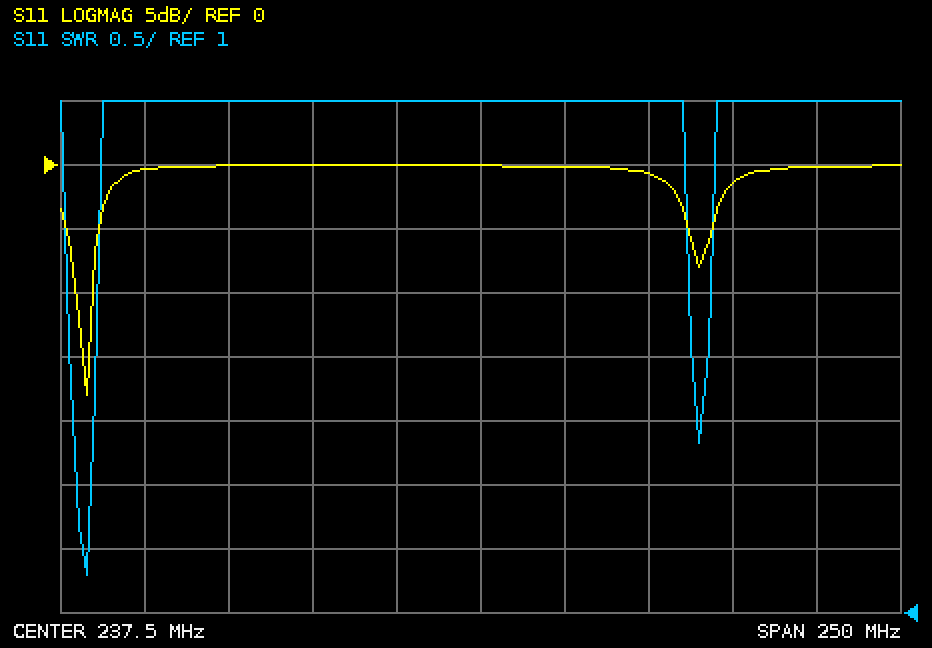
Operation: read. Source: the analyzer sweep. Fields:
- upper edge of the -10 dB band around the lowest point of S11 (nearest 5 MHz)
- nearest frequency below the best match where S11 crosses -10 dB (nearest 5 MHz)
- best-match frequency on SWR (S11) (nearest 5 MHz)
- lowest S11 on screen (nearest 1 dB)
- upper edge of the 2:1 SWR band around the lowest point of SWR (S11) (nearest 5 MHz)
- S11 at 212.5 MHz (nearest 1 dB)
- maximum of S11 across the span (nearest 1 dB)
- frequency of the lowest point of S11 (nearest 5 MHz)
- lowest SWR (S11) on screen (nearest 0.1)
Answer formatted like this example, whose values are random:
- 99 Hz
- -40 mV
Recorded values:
- 120 MHz
- 115 MHz
- 120 MHz
- -18 dB
- 120 MHz
- 0 dB
- 0 dB
- 120 MHz
- 1.3
